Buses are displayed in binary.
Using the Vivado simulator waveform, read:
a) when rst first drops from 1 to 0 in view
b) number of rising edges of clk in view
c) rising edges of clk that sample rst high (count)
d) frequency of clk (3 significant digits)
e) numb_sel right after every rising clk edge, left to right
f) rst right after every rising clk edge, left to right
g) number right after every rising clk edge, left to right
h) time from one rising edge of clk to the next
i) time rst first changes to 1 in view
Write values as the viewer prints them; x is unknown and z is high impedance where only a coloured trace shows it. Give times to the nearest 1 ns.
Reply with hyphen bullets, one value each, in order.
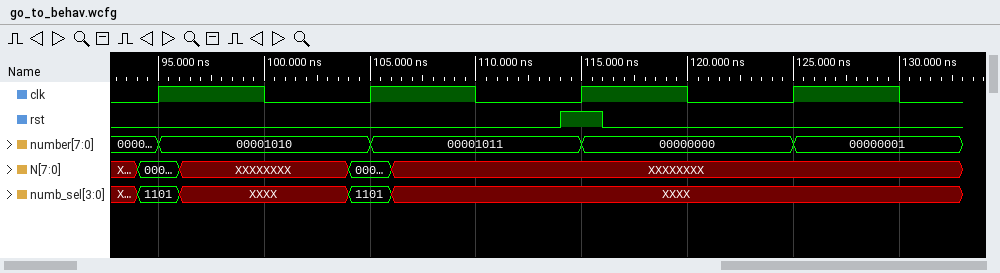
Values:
- 116 ns
- 4
- 1
- 100 MHz
- 1101, 1101, XXXX, XXXX
- 0 0 1 0
- 00001010, 00001011, 00000000, 00000001
- 10 ns
- 114 ns
